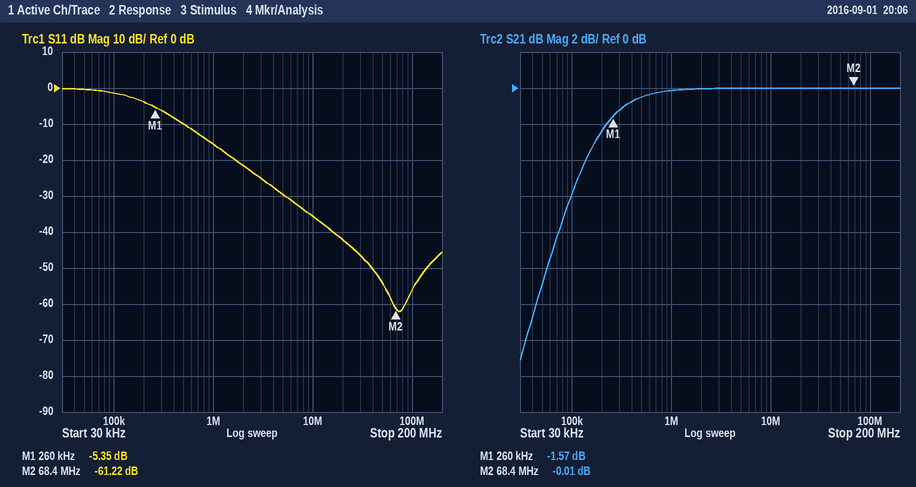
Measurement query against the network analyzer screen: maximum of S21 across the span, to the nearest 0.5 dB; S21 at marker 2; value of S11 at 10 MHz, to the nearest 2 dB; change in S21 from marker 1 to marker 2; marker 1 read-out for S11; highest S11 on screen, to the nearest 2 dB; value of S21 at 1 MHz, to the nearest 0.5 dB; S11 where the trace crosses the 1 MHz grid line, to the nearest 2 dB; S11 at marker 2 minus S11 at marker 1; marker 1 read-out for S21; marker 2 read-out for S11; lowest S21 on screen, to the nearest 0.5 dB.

0.0 dB
-0.01 dB
-36 dB
1.56 dB
-5.35 dB
0 dB
0.0 dB
-16 dB
-55.87 dB
-1.57 dB
-61.22 dB
-15.0 dB
